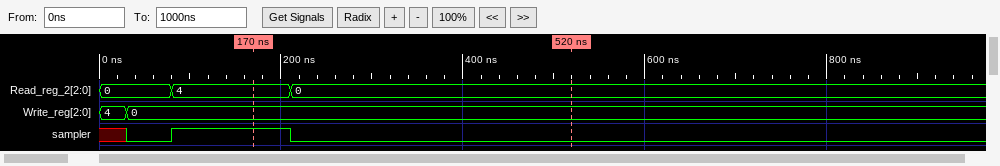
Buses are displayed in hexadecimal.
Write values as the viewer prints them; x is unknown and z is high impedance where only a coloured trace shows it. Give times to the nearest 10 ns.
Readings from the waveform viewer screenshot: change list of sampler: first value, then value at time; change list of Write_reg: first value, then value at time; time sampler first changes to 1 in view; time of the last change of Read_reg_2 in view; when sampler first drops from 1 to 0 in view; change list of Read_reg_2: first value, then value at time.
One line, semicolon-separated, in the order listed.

x, 0 at 30 ns, 1 at 80 ns, 0 at 210 ns; 4, 0 at 30 ns; 80 ns; 210 ns; 210 ns; 0, 4 at 80 ns, 0 at 210 ns
